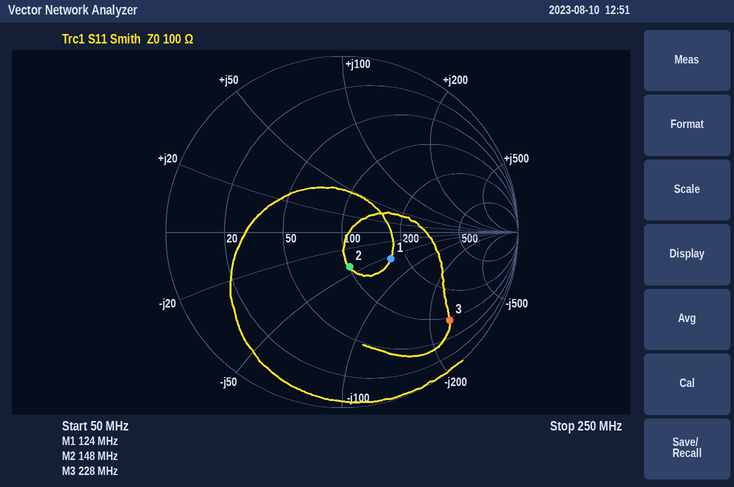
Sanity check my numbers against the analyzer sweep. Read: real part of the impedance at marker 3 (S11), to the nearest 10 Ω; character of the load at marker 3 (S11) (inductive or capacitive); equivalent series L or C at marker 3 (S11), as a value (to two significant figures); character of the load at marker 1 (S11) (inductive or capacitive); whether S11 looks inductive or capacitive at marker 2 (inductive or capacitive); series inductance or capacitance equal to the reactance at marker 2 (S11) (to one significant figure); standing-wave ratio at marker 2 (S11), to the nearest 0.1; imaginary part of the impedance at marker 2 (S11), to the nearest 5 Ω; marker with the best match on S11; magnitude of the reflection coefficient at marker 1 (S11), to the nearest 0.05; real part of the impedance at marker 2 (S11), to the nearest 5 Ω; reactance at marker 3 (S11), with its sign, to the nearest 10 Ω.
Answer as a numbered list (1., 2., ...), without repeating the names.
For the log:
1. 90 Ω
2. capacitive
3. 2.8 pF
4. capacitive
5. capacitive
6. 30 pF
7. 1.5
8. -40 Ω
9. marker 2
10. 0.30
11. 100 Ω
12. -250 Ω
